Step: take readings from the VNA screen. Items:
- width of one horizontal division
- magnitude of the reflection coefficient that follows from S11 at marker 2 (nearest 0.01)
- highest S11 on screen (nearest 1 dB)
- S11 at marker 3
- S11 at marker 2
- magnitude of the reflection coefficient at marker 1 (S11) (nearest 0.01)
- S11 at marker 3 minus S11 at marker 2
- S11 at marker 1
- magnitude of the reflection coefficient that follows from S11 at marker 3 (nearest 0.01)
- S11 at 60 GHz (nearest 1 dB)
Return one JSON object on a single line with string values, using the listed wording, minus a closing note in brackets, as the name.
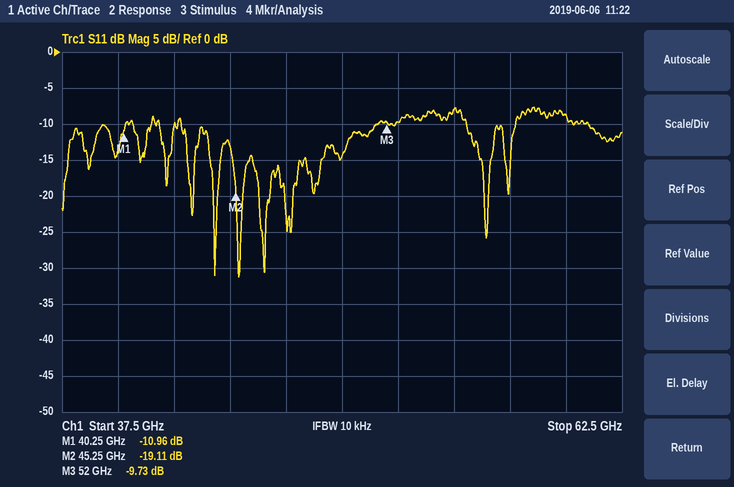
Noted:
{"width of one horizontal division": "2.5 GHz", "magnitude of the reflection coefficient that follows from S11 at marker 2": "0.11", "highest S11 on screen": "-8 dB", "S11 at marker 3": "-9.73 dB", "S11 at marker 2": "-19.11 dB", "magnitude of the reflection coefficient at marker 1 (S11)": "0.28", "S11 at marker 3 minus S11 at marker 2": "9.38 dB", "S11 at marker 1": "-10.96 dB", "magnitude of the reflection coefficient that follows from S11 at marker 3": "0.33", "S11 at 60 GHz": "-9 dB"}
